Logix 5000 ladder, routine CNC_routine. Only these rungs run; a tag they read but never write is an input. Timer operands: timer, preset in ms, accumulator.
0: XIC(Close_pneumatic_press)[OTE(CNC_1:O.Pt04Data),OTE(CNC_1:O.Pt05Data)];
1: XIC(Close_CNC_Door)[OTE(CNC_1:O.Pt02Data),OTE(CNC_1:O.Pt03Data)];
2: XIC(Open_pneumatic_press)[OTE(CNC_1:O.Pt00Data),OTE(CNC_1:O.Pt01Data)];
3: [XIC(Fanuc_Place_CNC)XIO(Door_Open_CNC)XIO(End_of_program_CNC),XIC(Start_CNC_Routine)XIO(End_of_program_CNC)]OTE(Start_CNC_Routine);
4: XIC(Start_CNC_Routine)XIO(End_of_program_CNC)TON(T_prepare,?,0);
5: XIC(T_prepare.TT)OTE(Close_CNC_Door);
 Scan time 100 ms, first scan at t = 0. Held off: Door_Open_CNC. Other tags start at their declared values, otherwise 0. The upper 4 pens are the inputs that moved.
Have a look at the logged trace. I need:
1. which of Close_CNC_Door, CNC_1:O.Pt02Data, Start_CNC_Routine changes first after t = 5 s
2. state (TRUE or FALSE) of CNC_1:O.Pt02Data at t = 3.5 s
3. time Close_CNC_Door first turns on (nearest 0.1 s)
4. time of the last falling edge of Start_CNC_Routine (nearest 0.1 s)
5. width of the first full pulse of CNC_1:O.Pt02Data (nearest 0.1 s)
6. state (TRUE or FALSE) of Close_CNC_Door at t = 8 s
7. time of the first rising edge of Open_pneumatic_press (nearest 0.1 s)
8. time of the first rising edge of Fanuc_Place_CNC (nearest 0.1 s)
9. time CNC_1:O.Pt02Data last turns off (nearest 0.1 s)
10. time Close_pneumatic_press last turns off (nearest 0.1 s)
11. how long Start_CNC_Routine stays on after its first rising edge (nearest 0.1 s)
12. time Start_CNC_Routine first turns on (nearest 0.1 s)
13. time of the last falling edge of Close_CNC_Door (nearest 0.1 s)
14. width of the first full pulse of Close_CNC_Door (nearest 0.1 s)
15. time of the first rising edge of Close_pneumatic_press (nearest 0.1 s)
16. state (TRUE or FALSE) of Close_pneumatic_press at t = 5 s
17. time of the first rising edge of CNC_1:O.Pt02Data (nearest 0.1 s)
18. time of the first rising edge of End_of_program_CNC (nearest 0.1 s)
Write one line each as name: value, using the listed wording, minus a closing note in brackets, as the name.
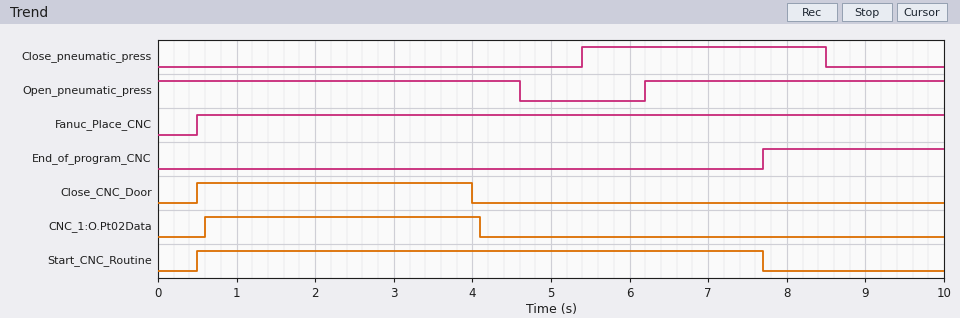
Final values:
which of Close_CNC_Door, CNC_1:O.Pt02Data, Start_CNC_Routine changes first after t = 5 s: Start_CNC_Routine
state (TRUE or FALSE) of CNC_1:O.Pt02Data at t = 3.5 s: TRUE
time Close_CNC_Door first turns on: 0.5 s
time of the last falling edge of Start_CNC_Routine: 7.7 s
width of the first full pulse of CNC_1:O.Pt02Data: 3.5 s
state (TRUE or FALSE) of Close_CNC_Door at t = 8 s: FALSE
time of the first rising edge of Open_pneumatic_press: 6.2 s
time of the first rising edge of Fanuc_Place_CNC: 0.5 s
time CNC_1:O.Pt02Data last turns off: 4.1 s
time Close_pneumatic_press last turns off: 8.5 s
how long Start_CNC_Routine stays on after its first rising edge: 7.2 s
time Start_CNC_Routine first turns on: 0.5 s
time of the last falling edge of Close_CNC_Door: 4.0 s
width of the first full pulse of Close_CNC_Door: 3.5 s
time of the first rising edge of Close_pneumatic_press: 5.4 s
state (TRUE or FALSE) of Close_pneumatic_press at t = 5 s: FALSE
time of the first rising edge of CNC_1:O.Pt02Data: 0.6 s
time of the first rising edge of End_of_program_CNC: 7.7 s
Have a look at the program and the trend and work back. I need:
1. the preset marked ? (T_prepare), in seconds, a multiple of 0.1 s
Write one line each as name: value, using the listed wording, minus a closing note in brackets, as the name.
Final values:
the preset marked ? (T_prepare), in seconds, a multiple of 0.1 s: 3.5 s
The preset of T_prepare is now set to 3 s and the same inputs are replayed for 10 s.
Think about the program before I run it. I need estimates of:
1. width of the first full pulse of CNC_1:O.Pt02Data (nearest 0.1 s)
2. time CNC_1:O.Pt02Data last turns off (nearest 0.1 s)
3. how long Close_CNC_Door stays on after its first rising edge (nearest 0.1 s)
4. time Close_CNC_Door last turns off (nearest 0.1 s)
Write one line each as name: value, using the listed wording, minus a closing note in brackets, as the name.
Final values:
width of the first full pulse of CNC_1:O.Pt02Data: 3.0 s
time CNC_1:O.Pt02Data last turns off: 3.6 s
how long Close_CNC_Door stays on after its first rising edge: 3.0 s
time Close_CNC_Door last turns off: 3.5 s
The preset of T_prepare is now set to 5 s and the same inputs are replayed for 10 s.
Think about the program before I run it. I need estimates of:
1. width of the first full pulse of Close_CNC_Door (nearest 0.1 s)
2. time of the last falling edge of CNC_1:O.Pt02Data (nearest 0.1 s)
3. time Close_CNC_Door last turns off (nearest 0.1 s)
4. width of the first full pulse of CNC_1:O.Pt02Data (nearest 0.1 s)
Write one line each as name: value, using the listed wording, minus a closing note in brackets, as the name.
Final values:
width of the first full pulse of Close_CNC_Door: 5.0 s
time of the last falling edge of CNC_1:O.Pt02Data: 5.6 s
time Close_CNC_Door last turns off: 5.5 s
width of the first full pulse of CNC_1:O.Pt02Data: 5.0 s
